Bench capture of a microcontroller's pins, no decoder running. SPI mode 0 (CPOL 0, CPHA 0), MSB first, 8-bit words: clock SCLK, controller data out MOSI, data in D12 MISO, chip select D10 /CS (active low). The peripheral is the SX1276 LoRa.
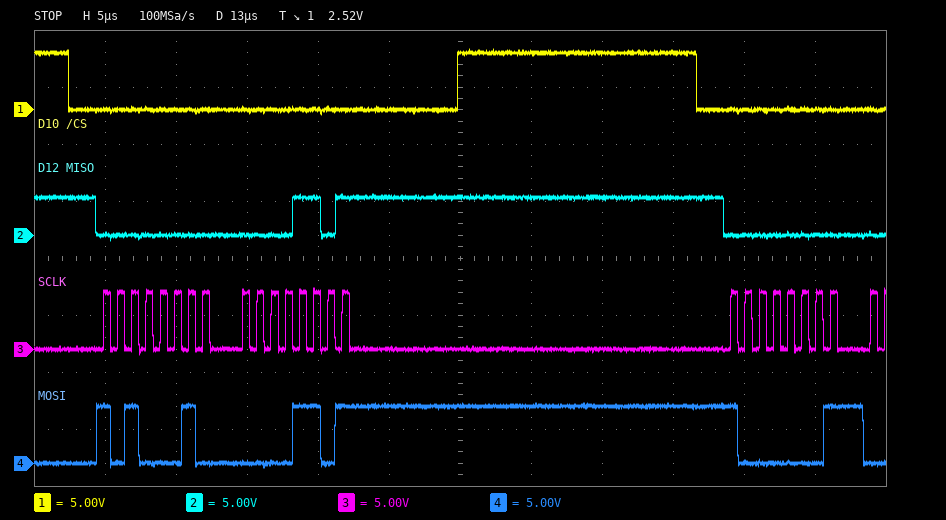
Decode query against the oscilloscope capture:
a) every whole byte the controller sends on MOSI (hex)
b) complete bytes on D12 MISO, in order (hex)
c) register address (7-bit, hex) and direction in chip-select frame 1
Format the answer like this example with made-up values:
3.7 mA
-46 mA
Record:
0xA2 0x0D 0x81
0x00 0x0D 0x00
0x22 write
